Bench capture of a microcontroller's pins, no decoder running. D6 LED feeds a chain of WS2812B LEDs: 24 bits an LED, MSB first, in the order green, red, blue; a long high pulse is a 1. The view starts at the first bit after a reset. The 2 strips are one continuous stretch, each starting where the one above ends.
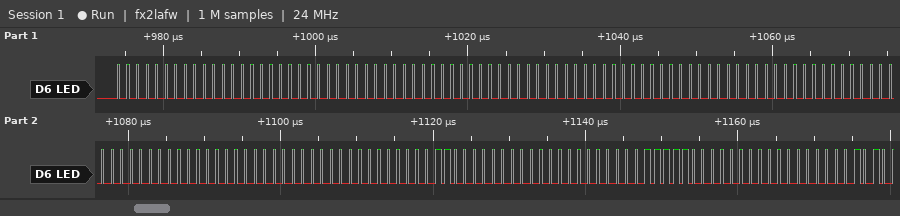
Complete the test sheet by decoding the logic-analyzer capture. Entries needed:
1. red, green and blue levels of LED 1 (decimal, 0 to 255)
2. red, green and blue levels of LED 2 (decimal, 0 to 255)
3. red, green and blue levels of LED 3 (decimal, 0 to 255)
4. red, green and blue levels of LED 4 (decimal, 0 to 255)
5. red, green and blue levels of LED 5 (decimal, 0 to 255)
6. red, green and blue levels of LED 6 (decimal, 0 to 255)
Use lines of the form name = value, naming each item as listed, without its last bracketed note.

red, green and blue levels of LED 1 = 0, 0, 0
red, green and blue levels of LED 2 = 0, 0, 0
red, green and blue levels of LED 3 = 0, 0, 0
red, green and blue levels of LED 4 = 0, 0, 0
red, green and blue levels of LED 5 = 0, 0, 6
red, green and blue levels of LED 6 = 0, 0, 31
